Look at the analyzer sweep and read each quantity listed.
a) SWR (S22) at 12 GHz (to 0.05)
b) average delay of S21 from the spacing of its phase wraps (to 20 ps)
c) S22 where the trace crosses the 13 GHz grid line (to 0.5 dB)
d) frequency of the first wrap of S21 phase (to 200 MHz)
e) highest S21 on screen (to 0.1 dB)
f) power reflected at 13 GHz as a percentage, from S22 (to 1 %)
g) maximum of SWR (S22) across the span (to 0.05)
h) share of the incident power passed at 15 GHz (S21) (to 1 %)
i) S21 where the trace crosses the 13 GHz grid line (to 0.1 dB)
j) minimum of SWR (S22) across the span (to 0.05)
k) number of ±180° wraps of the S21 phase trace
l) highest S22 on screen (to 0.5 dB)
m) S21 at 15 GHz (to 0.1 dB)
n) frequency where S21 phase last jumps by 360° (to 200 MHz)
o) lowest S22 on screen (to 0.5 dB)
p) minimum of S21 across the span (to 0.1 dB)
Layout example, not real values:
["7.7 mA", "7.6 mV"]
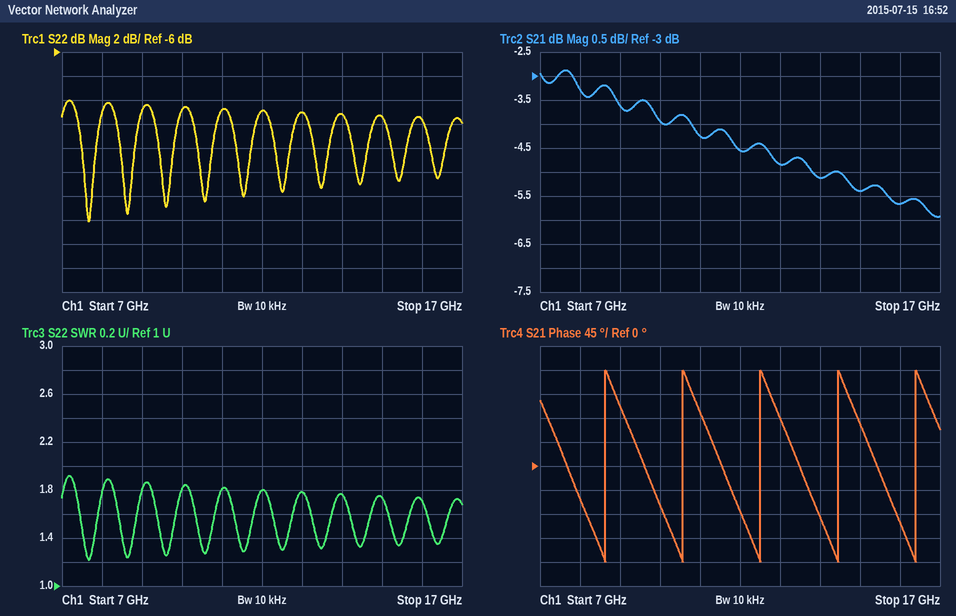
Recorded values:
["1.80", "520 ps", "-11.0 dB", "8.6 GHz", "-2.9 dB", "8 %", "1.90", "29 %", "-4.8 dB", "1.20", "5", "-10.0 dB", "-5.4 dB", "16.4 GHz", "-20.0 dB", "-5.9 dB"]
